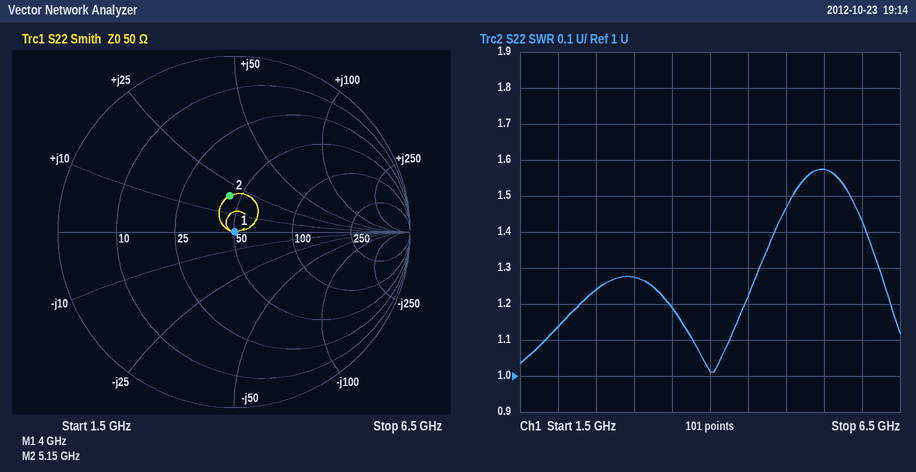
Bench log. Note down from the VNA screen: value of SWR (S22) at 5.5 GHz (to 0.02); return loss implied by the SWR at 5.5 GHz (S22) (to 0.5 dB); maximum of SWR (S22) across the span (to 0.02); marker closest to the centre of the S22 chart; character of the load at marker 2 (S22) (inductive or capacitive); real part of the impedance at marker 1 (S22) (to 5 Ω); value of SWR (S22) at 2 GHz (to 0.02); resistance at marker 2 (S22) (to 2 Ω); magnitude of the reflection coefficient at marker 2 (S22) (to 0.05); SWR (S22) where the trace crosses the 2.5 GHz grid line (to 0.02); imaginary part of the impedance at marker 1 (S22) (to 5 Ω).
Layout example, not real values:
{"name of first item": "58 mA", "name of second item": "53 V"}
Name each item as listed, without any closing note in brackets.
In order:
{"value of SWR (S22) at 5.5 GHz": "1.58", "return loss implied by the SWR at 5.5 GHz (S22)": "13.0 dB", "maximum of SWR (S22) across the span": "1.58", "marker closest to the centre of the S22 chart": "marker 1", "character of the load at marker 2 (S22)": "inductive", "real part of the impedance at marker 1 (S22)": "50 Ω", "value of SWR (S22) at 2 GHz": "1.14", "resistance at marker 2 (S22)": "44 Ω", "magnitude of the reflection coefficient at marker 2 (S22)": "0.20", "SWR (S22) where the trace crosses the 2.5 GHz grid line": "1.24", "imaginary part of the impedance at marker 1 (S22)": "0 Ω"}
